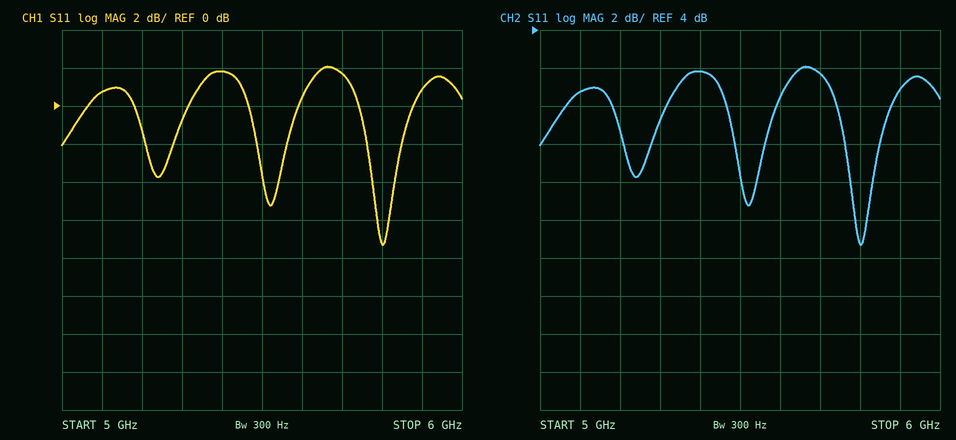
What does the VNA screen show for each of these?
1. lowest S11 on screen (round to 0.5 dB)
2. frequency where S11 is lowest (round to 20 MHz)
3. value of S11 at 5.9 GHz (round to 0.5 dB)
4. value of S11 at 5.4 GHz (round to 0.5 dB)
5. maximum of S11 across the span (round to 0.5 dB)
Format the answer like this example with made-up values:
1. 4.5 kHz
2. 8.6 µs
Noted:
1. -7.5 dB
2. 5.80 GHz
3. 1.0 dB
4. 2.0 dB
5. 2.0 dB
